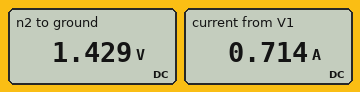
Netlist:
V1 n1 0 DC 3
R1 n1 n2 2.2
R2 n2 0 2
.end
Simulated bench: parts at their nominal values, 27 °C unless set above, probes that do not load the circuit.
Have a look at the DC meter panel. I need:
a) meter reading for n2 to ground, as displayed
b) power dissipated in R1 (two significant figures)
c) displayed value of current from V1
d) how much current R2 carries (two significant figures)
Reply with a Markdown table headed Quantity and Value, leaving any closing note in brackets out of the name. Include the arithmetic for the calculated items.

| Quantity | Value |
|---|---|
| meter reading for n2 to ground, as displayed | 1.429 V |
| power dissipated in R1 | (3 V - 1.429 V)^2 / 2.2 Ω = 1.1 W |
| displayed value of current from V1 | 0.714 A |
| how much current R2 carries | (1.429 V) / 2 Ω = 710 mA |
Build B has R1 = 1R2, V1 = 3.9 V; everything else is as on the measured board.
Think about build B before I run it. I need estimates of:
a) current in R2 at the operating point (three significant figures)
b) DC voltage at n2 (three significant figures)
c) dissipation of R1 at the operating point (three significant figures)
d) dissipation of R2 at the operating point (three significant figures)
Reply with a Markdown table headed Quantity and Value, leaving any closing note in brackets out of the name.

| Quantity | Value |
|---|---|
| current in R2 at the operating point | 1.22 A |
| DC voltage at n2 | 2.44 V |
| dissipation of R1 at the operating point | 1.78 W |
| dissipation of R2 at the operating point | 2.97 W |
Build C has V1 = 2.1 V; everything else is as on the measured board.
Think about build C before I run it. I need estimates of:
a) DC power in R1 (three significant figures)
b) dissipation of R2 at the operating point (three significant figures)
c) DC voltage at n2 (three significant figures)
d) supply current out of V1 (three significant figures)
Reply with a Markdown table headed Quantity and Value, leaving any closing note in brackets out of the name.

| Quantity | Value |
|---|---|
| DC power in R1 | 550 mW |
| dissipation of R2 at the operating point | 500 mW |
| DC voltage at n2 | 1.00 V |
| supply current out of V1 | 500 mA |
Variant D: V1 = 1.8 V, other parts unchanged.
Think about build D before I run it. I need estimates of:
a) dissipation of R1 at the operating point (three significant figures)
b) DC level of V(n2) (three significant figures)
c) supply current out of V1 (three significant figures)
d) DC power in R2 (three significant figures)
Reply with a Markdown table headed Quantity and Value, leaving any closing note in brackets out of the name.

| Quantity | Value |
|---|---|
| dissipation of R1 at the operating point | 404 mW |
| DC level of V(n2) | 857 mV |
| supply current out of V1 | 429 mA |
| DC power in R2 | 367 mW |
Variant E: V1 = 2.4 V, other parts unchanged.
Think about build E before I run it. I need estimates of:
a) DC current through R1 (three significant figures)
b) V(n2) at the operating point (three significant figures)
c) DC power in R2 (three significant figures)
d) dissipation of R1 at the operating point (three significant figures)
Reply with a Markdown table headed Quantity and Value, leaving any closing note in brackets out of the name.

| Quantity | Value |
|---|---|
| DC current through R1 | 571 mA |
| V(n2) at the operating point | 1.14 V |
| DC power in R2 | 653 mW |
| dissipation of R1 at the operating point | 718 mW |
